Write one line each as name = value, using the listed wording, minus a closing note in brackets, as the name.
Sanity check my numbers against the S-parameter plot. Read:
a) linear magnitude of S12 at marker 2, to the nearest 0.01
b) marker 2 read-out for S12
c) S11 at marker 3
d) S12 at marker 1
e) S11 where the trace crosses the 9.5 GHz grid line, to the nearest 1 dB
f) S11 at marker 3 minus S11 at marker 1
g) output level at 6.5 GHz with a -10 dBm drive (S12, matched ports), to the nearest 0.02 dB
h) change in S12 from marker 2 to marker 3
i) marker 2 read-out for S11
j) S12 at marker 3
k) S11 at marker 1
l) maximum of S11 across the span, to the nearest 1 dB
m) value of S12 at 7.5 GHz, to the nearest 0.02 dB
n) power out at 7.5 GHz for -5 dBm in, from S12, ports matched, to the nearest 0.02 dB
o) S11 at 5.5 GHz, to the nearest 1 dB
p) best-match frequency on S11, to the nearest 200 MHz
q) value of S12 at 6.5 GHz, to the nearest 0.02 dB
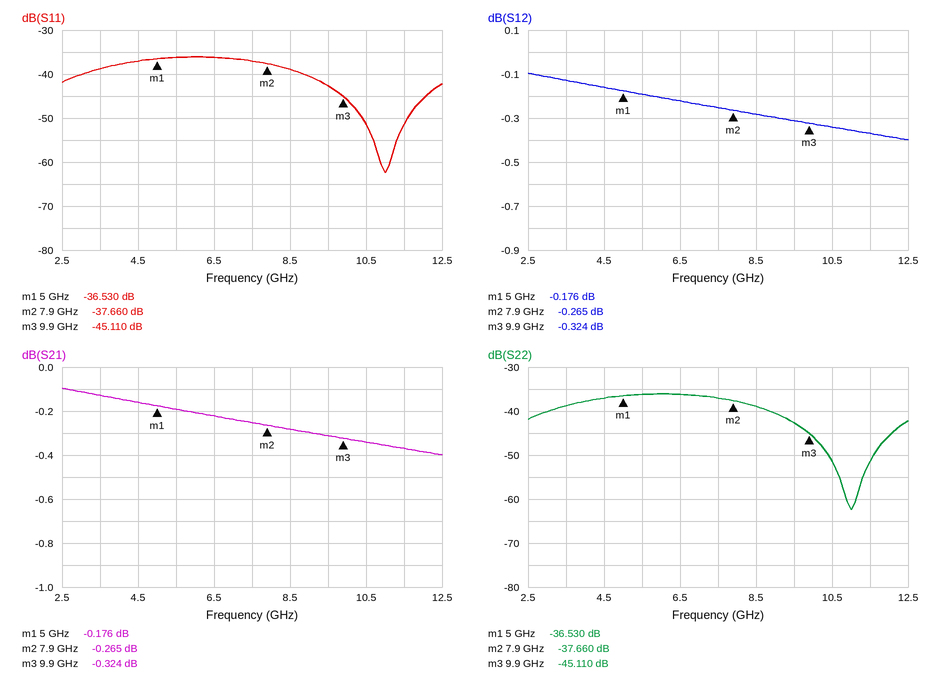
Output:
linear magnitude of S12 at marker 2, to the nearest 0.01 = 0.97
marker 2 read-out for S12 = -0.265 dB
S11 at marker 3 = -45.110 dB
S12 at marker 1 = -0.176 dB
S11 where the trace crosses the 9.5 GHz grid line, to the nearest 1 dB = -43 dB
S11 at marker 3 minus S11 at marker 1 = -8.580 dB
output level at 6.5 GHz with a -10 dBm drive (S12, matched ports), to the nearest 0.02 dB = -10.22 dBm
change in S12 from marker 2 to marker 3 = -0.059 dB
marker 2 read-out for S11 = -37.660 dB
S12 at marker 3 = -0.324 dB
S11 at marker 1 = -36.530 dB
maximum of S11 across the span, to the nearest 1 dB = -36 dB
value of S12 at 7.5 GHz, to the nearest 0.02 dB = -0.26 dB
power out at 7.5 GHz for -5 dBm in, from S12, ports matched, to the nearest 0.02 dB = -5.26 dBm
S11 at 5.5 GHz, to the nearest 1 dB = -36 dB
best-match frequency on S11, to the nearest 200 MHz = 11.0 GHz
value of S12 at 6.5 GHz, to the nearest 0.02 dB = -0.22 dB
